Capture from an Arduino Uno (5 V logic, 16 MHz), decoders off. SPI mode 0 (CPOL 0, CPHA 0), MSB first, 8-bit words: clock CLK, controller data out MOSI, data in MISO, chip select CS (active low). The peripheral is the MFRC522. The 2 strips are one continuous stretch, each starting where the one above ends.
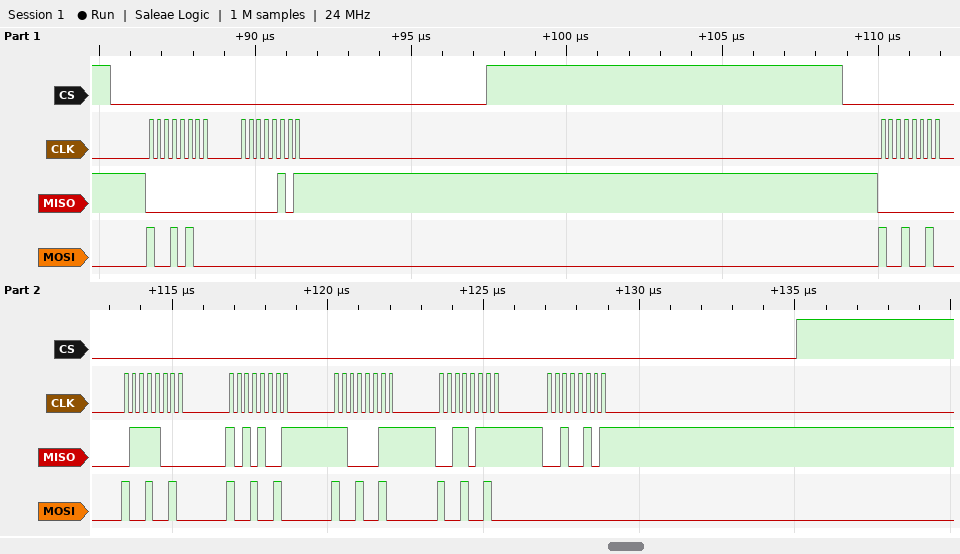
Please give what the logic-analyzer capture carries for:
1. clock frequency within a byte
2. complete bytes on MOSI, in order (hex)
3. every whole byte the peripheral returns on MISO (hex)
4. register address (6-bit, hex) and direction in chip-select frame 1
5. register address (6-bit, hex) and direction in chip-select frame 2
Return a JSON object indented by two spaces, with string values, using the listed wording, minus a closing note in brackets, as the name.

{
  "clock frequency within a byte": "4 MHz",
  "complete bytes on MOSI, in order": "94 00 92 92 92 92 92 00",
  "every whole byte the peripheral returns on MISO": "00 05 00 78 A9 C3 37 25",
  "register address (6-bit, hex) and direction in chip-select frame 1": "0x0A read",
  "register address (6-bit, hex) and direction in chip-select frame 2": "0x09 read"
}
